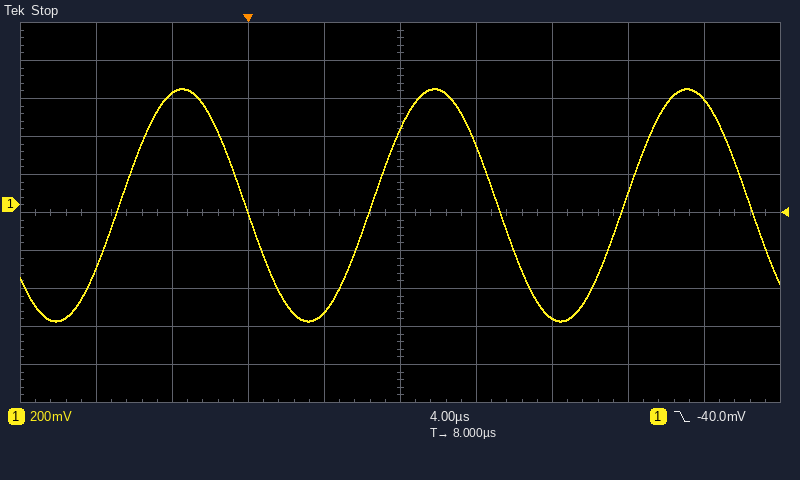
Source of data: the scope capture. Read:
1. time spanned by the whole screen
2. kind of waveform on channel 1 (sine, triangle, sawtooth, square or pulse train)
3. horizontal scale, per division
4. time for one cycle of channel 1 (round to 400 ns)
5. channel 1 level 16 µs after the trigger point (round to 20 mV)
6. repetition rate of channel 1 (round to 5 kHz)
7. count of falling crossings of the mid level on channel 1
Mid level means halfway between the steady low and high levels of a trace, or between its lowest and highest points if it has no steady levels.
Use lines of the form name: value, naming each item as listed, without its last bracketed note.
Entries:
time spanned by the whole screen: 40 µs
kind of waveform on channel 1: sine
horizontal scale, per division: 4 µs
time for one cycle of channel 1: 13.2 µs
channel 1 level 16 µs after the trigger point: -600 mV
repetition rate of channel 1: 75 kHz
count of falling crossings of the mid level on channel 1: 3
